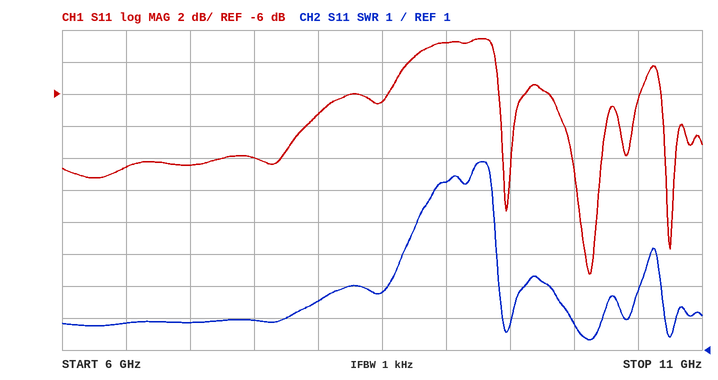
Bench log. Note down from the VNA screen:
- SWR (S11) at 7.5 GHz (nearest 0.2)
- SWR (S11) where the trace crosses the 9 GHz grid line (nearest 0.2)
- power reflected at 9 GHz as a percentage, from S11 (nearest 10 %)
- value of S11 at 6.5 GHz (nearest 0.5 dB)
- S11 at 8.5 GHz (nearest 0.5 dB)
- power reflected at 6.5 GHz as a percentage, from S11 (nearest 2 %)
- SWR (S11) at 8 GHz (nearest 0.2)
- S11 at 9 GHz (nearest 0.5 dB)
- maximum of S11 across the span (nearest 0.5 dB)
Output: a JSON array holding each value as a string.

["2.0", "6.2", "50 %", "-10.5 dB", "-6.5 dB", "8 %", "2.6", "-3.0 dB", "-2.5 dB"]
